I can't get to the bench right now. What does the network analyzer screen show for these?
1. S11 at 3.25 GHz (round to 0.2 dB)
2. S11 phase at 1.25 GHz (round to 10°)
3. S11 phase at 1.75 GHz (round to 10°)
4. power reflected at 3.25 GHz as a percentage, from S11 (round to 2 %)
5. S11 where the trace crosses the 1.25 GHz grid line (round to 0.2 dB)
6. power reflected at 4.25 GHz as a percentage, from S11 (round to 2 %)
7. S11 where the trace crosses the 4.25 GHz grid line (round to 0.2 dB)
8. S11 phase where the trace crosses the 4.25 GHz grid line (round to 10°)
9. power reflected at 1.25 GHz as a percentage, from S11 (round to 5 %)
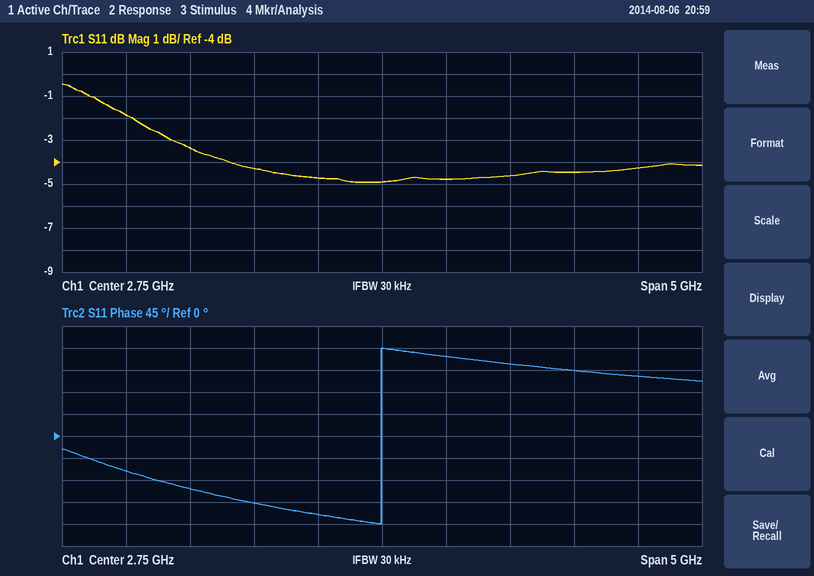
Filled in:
-4.8 dB
-110°
-140°
34 %
-3.4 dB
36 %
-4.4 dB
130°
45 %
